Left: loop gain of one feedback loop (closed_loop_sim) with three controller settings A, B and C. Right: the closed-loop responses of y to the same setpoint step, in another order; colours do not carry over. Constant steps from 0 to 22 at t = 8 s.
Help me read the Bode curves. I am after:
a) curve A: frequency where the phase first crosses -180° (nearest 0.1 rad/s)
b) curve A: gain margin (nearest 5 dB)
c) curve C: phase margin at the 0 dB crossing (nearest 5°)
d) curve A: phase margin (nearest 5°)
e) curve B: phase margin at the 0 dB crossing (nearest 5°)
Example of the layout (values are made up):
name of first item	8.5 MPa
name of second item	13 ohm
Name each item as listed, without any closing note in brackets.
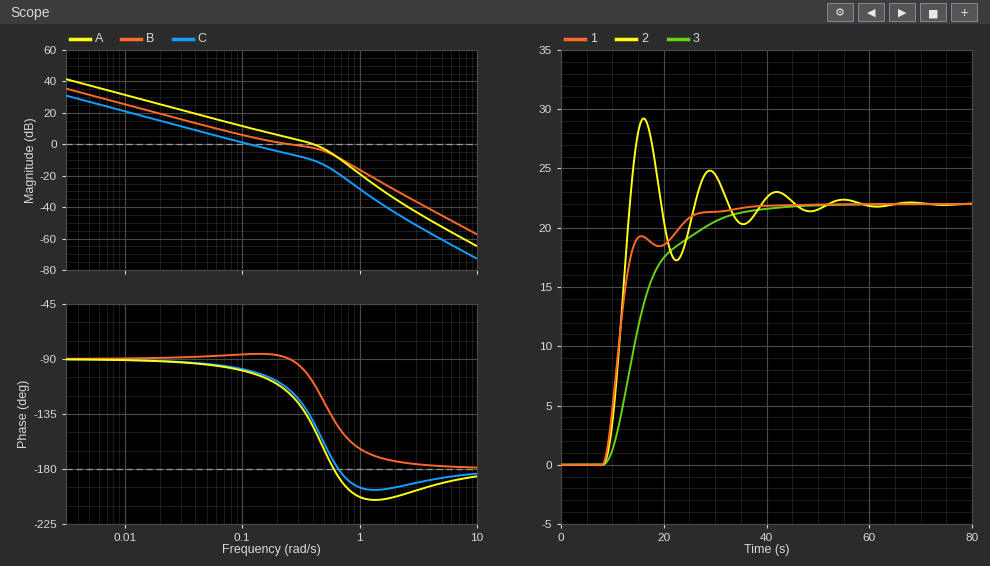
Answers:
curve A: frequency where the phase first crosses -180°	0.6 rad/s
curve A: gain margin	5 dB
curve C: phase margin at the 0 dB crossing	80°
curve A: phase margin	35°
curve B: phase margin at the 0 dB crossing	90°
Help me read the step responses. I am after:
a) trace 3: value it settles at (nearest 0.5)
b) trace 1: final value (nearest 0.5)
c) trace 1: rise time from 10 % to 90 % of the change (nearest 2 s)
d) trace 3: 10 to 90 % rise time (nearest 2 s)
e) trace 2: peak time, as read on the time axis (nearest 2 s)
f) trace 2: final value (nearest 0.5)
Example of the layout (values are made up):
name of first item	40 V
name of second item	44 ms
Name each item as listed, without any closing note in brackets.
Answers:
trace 3: value it settles at	22.0
trace 1: final value	22.0
trace 1: rise time from 10 % to 90 % of the change	14 s
trace 3: 10 to 90 % rise time	16 s
trace 2: peak time, as read on the time axis	16 s
trace 2: final value	22.0
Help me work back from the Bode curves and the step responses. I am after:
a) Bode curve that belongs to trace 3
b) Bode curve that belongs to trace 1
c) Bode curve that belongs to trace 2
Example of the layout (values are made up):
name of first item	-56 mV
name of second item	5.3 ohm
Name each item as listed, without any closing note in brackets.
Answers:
Bode curve that belongs to trace 3	C
Bode curve that belongs to trace 1	B
Bode curve that belongs to trace 2	A
